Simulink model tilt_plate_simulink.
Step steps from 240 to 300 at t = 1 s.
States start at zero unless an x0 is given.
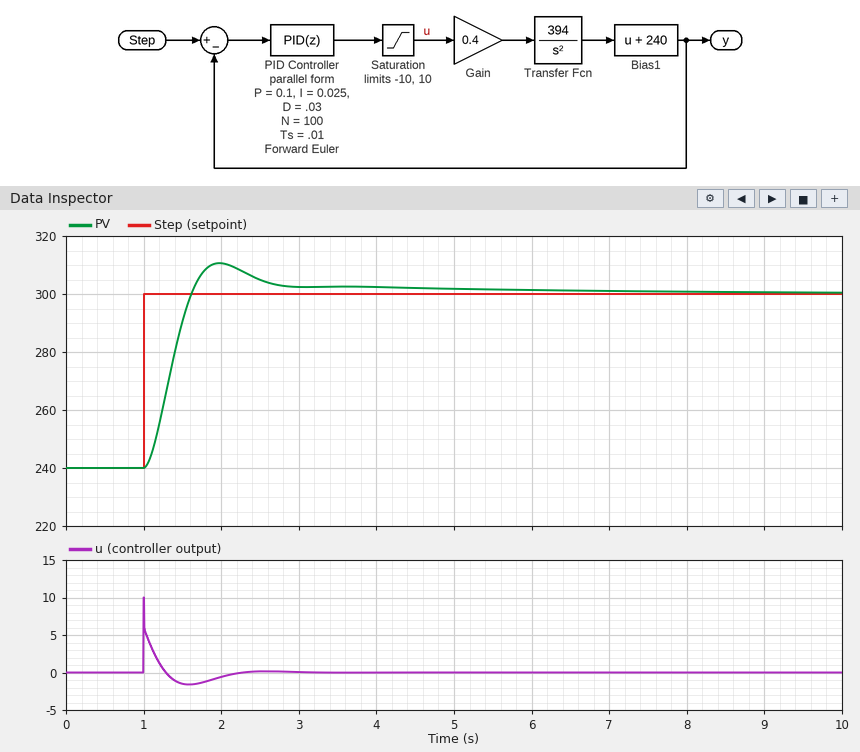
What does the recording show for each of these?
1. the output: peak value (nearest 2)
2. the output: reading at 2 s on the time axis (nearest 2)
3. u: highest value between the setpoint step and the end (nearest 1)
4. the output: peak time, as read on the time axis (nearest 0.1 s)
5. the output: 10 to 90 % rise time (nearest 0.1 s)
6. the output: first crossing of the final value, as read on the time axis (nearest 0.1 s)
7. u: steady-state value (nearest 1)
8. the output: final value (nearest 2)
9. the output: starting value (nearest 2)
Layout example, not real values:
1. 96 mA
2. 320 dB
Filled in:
1. 310
2. 310
3. 10
4. 2.0 s
5. 0.4 s
6. 1.6 s
7. 0
8. 300
9. 240
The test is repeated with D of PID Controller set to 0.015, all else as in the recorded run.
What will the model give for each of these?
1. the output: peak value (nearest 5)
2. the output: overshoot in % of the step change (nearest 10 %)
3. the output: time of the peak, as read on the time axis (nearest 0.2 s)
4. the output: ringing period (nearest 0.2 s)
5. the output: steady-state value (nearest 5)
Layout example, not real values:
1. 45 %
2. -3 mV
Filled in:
1. 330
2. 50 %
3. 1.8 s
4. 1.6 s
5. 300
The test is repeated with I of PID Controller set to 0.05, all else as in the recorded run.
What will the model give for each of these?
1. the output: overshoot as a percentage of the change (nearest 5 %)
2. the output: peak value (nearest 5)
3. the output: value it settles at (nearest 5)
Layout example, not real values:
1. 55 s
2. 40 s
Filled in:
1. 25 %
2. 315
3. 300
